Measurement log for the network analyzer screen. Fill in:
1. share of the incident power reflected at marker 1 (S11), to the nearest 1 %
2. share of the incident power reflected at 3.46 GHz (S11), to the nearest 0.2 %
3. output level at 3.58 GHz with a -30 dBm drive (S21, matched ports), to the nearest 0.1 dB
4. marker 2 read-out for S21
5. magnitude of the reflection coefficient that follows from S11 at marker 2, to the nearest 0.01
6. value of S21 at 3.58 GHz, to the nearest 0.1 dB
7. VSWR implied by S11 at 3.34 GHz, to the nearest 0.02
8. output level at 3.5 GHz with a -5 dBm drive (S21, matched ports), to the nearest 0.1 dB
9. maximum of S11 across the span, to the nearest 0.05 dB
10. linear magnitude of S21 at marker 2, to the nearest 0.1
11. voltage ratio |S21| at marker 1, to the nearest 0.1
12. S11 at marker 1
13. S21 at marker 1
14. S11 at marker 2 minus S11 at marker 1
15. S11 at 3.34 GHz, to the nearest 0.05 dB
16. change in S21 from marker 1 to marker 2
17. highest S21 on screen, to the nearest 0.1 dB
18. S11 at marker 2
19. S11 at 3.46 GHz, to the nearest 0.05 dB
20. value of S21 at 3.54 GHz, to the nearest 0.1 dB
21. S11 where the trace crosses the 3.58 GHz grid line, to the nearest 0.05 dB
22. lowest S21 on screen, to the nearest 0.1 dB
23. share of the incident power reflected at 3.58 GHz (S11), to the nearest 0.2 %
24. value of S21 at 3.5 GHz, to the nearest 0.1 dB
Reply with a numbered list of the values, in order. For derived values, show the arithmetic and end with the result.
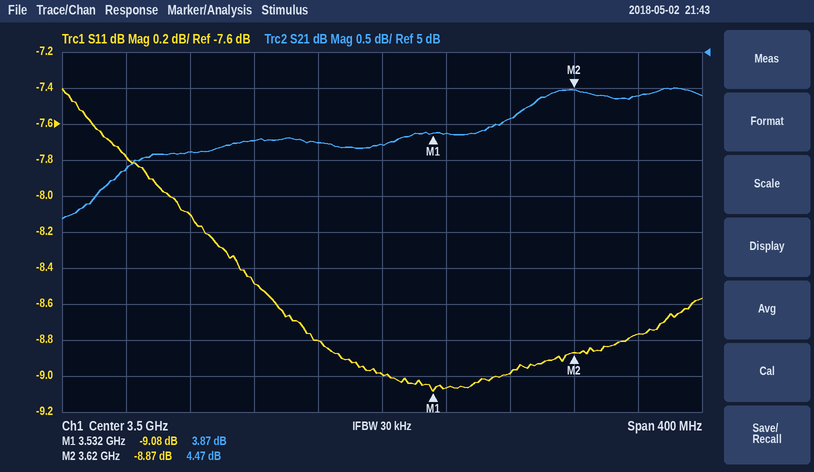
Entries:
1. 10^(-9.08/10) ≈ 12 %
2. 10^(-8.8/10) ≈ 13.2 %
3. -30 dBm + (4.1 dB) = -25.9 dBm
4. 4.47 dB
5. 10^(-8.87/20) ≈ 0.36
6. 4.1 dB
7. |Γ| = 10^(-7.8/20) = 0.4074; VSWR = (1 + 0.4074)/(1 − 0.4074) ≈ 2.37, so 2.38 to the nearest 0.02
8. -5 dBm + (3.7 dB) = -1.3 dBm
9. -7.40 dB
10. 10^(4.47/20) ≈ 1.7
11. 10^(3.87/20) ≈ 1.6
12. -9.08 dB
13. 3.87 dB
14. -8.87 − (-9.08) = 0.21 dB
15. -7.80 dB
16. 4.47 − (3.87) = 0.60 dB
17. 4.5 dB
18. -8.87 dB
19. -8.80 dB
20. 3.9 dB
21. -9.00 dB
22. 2.7 dB
23. 10^(-9/10) ≈ 12.6 %
24. 3.7 dB
